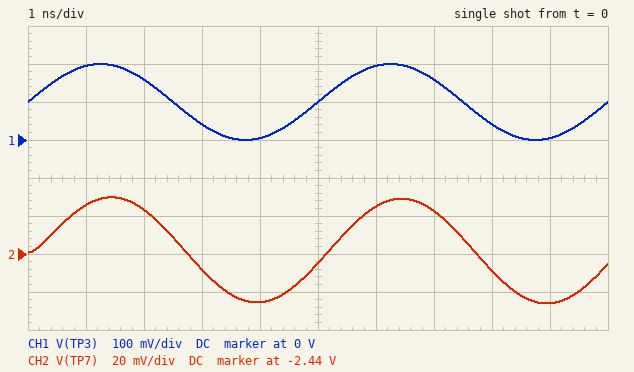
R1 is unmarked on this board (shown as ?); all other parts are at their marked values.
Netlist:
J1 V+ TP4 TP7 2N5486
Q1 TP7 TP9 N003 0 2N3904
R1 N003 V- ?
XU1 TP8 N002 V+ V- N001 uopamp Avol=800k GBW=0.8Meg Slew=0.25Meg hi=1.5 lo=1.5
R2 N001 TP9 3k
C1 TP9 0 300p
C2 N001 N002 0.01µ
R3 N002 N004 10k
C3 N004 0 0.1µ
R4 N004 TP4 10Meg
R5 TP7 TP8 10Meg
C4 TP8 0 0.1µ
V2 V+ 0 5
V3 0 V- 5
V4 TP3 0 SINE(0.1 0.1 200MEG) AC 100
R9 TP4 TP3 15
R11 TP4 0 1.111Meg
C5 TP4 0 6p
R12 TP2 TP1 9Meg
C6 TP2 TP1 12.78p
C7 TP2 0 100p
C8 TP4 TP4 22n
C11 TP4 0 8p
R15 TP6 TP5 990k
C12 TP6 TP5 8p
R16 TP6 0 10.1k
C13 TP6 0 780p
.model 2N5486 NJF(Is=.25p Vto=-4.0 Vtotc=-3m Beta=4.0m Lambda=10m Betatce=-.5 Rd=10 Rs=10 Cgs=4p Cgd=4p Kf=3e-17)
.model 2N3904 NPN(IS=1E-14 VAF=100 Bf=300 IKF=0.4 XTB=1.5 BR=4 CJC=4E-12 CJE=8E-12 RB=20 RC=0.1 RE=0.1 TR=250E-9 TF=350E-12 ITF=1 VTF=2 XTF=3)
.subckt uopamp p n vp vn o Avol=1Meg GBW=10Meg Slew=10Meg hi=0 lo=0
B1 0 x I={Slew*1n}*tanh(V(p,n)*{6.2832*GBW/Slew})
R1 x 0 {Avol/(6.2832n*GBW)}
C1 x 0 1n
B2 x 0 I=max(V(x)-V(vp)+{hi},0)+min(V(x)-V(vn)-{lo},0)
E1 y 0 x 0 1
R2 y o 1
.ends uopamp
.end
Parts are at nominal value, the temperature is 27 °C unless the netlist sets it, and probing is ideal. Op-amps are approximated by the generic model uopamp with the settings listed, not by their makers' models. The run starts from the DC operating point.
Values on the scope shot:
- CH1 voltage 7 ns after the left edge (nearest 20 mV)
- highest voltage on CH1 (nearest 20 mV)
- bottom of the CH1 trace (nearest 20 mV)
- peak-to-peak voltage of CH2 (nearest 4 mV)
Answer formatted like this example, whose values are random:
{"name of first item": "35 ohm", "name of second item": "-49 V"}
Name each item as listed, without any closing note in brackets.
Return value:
{"CH1 voltage 7 ns after the left edge": "160 mV", "highest voltage on CH1": "200 mV", "bottom of the CH1 trace": "0 V", "peak-to-peak voltage of CH2": "56 mV"}
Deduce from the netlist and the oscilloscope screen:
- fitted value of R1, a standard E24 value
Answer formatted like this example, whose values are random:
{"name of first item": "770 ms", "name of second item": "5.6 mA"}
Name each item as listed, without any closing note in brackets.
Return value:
{"fitted value of R1, a standard E24 value": "18 Ω"}
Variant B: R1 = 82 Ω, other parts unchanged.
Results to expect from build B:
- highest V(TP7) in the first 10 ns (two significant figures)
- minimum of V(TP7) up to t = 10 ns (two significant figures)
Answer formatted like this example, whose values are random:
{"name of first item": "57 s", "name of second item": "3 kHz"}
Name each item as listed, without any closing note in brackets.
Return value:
{"highest V(TP7) in the first 10 ns": "430 mV", "minimum of V(TP7) up to t = 10 ns": "250 mV"}
